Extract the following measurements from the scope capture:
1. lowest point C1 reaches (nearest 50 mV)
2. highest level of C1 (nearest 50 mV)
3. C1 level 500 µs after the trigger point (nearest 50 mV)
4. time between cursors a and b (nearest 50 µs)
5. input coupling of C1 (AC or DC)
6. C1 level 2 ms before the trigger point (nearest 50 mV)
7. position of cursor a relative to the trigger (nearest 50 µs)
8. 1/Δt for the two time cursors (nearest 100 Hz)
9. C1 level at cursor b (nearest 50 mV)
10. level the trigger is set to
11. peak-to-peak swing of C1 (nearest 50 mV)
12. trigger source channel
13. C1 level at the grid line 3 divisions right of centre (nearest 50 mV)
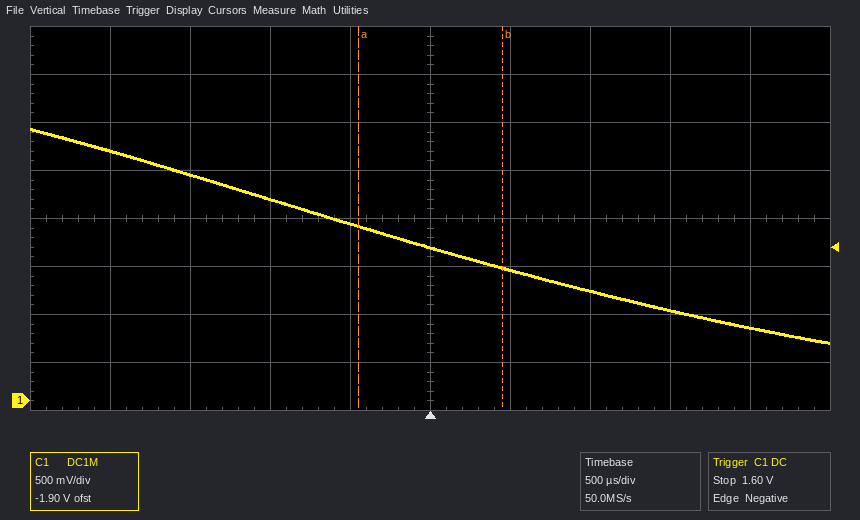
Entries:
600 mV
2.85 V
1.35 V
900 µs
DC
2.60 V
-450 µs
1.1 kHz
1.40 V
1.60 V
2.25 V
C1
950 mV
